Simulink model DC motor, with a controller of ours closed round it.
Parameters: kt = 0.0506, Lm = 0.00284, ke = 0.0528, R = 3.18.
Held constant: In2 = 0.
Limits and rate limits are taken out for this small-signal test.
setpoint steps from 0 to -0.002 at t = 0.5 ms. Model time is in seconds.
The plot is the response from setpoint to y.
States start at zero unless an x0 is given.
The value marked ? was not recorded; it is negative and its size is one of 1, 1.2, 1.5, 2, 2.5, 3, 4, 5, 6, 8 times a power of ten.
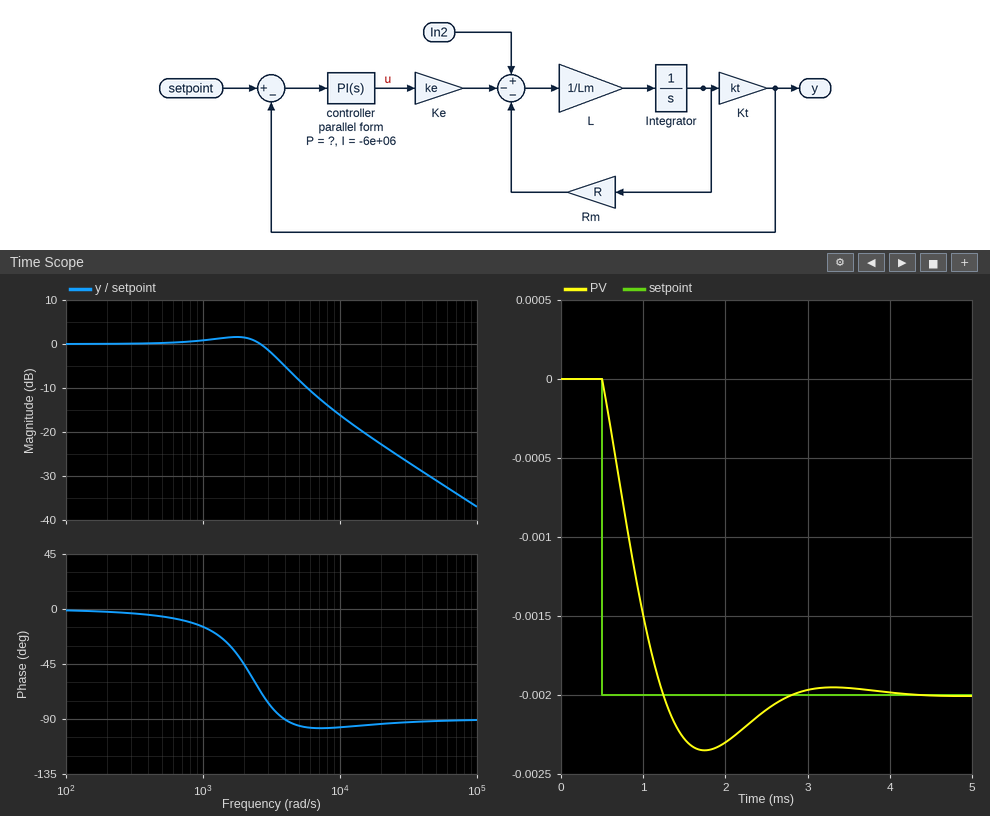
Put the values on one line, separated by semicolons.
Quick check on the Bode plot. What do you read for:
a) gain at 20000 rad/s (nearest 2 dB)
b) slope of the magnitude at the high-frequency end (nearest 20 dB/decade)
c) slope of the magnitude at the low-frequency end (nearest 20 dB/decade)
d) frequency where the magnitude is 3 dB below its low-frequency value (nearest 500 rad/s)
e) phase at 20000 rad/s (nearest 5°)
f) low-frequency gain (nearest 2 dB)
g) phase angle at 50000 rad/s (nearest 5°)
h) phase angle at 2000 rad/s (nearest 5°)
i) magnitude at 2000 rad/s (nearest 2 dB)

-22 dB; -20 dB/decade; 0 dB/decade; 3500 rad/s; -95°; 0 dB; -90°; -45°; 2 dB
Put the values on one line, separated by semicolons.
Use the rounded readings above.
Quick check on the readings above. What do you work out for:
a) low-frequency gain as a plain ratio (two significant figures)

1.0
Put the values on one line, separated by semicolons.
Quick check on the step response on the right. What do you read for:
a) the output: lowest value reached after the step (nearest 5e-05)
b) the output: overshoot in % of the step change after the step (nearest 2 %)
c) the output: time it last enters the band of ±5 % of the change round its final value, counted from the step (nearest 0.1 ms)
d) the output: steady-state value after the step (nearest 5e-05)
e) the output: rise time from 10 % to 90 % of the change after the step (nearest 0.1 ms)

-0.00235; 18 %; 2.0 ms; -0.00200; 0.6 ms
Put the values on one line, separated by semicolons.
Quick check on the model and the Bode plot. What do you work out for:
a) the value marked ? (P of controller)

-1500
